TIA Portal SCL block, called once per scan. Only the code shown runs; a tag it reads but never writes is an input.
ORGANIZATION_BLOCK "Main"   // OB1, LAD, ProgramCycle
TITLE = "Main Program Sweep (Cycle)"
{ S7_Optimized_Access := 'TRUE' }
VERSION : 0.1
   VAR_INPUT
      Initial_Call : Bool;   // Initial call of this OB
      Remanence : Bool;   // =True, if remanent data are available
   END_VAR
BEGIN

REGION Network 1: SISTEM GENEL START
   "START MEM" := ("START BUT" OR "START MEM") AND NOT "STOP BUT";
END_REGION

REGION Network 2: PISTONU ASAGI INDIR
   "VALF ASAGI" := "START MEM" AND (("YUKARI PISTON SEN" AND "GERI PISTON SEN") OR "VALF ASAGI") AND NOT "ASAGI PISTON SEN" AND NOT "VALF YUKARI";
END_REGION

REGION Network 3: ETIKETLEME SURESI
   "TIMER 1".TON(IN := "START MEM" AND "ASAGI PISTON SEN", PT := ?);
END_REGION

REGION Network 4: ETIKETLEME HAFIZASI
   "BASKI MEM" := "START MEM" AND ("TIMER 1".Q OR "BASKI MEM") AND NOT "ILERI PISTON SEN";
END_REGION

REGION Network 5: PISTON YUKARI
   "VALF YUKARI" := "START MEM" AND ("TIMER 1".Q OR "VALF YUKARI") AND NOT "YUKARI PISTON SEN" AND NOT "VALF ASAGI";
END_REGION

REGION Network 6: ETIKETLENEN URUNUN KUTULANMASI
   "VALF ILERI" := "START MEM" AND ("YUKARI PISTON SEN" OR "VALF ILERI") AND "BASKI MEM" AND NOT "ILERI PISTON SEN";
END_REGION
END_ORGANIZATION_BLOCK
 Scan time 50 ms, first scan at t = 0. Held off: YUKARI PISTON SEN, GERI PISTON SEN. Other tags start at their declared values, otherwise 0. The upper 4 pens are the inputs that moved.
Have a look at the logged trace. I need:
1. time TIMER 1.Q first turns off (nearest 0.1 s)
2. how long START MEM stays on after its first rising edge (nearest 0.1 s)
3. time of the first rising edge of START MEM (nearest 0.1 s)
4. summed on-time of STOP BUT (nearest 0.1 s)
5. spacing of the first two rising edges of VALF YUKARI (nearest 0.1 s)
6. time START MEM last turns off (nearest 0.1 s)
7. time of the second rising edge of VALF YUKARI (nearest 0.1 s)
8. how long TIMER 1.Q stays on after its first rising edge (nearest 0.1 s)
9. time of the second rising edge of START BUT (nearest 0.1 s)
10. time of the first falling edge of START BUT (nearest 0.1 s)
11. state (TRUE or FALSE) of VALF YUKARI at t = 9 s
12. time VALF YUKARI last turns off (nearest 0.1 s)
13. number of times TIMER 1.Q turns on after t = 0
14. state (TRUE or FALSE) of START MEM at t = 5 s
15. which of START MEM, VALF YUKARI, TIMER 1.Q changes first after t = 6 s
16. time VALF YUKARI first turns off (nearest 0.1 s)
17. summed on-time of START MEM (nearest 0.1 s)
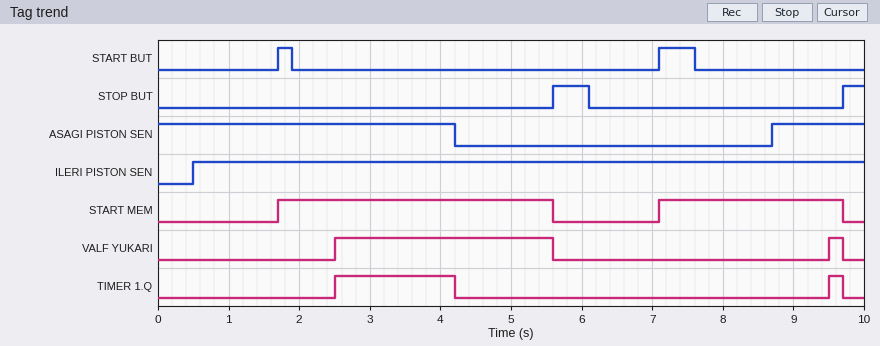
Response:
4.2 s
3.9 s
1.7 s
0.8 s
7.0 s
9.7 s
9.5 s
1.7 s
7.1 s
1.9 s
FALSE
9.7 s
2
TRUE
START MEM
5.6 s
6.5 s
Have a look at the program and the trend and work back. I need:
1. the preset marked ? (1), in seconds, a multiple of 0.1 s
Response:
0.8 s
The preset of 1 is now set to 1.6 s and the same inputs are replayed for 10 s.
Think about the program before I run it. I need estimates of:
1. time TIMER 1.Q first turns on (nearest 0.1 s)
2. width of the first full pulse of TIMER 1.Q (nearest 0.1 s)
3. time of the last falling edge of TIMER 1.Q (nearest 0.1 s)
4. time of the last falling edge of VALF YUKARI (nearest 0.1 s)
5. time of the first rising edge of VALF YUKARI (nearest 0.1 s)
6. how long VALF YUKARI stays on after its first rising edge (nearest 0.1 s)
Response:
3.3 s
0.9 s
4.2 s
5.6 s
3.3 s
2.3 s
